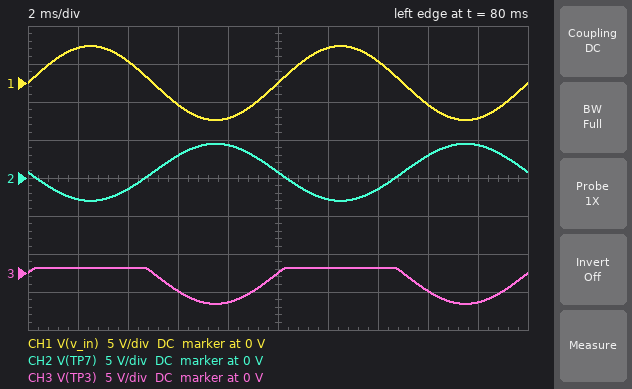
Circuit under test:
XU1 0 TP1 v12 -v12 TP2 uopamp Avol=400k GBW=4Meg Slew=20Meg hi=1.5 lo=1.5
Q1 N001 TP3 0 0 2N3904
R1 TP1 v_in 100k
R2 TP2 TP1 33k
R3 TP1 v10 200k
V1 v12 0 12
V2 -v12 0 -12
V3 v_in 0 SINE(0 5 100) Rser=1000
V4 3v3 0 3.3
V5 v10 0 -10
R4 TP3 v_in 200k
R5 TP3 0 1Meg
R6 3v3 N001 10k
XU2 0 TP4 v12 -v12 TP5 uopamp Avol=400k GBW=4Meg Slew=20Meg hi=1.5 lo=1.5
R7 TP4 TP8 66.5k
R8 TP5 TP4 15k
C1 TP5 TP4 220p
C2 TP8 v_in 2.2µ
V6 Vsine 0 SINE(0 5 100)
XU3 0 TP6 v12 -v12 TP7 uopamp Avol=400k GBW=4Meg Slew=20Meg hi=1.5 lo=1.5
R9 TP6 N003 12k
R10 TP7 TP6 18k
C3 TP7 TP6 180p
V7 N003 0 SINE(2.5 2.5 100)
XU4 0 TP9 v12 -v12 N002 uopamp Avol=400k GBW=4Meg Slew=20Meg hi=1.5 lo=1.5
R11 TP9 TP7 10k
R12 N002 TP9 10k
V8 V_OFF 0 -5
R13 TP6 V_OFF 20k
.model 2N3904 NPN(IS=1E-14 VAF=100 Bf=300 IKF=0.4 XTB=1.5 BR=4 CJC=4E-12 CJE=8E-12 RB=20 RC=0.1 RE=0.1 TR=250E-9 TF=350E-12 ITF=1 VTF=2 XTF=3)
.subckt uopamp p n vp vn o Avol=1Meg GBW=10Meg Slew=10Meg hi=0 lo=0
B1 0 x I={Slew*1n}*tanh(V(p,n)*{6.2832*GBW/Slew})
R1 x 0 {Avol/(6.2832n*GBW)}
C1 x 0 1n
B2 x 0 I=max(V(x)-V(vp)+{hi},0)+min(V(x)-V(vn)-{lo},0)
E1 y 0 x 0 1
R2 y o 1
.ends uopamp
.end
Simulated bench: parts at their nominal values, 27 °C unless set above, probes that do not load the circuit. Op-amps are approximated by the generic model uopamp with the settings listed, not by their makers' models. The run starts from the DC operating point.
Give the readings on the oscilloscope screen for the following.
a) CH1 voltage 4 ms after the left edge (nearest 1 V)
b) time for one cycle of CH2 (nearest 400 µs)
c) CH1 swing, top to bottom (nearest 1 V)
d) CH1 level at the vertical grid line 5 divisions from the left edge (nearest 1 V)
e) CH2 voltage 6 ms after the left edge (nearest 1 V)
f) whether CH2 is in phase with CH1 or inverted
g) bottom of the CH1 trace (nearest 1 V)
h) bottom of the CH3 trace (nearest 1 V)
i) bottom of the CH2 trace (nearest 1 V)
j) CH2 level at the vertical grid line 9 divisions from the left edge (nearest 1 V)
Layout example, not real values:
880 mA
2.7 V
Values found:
3 V
10.0 ms
10 V
0 V
3 V
inverted
-5 V
-4 V
-3 V
4 V
